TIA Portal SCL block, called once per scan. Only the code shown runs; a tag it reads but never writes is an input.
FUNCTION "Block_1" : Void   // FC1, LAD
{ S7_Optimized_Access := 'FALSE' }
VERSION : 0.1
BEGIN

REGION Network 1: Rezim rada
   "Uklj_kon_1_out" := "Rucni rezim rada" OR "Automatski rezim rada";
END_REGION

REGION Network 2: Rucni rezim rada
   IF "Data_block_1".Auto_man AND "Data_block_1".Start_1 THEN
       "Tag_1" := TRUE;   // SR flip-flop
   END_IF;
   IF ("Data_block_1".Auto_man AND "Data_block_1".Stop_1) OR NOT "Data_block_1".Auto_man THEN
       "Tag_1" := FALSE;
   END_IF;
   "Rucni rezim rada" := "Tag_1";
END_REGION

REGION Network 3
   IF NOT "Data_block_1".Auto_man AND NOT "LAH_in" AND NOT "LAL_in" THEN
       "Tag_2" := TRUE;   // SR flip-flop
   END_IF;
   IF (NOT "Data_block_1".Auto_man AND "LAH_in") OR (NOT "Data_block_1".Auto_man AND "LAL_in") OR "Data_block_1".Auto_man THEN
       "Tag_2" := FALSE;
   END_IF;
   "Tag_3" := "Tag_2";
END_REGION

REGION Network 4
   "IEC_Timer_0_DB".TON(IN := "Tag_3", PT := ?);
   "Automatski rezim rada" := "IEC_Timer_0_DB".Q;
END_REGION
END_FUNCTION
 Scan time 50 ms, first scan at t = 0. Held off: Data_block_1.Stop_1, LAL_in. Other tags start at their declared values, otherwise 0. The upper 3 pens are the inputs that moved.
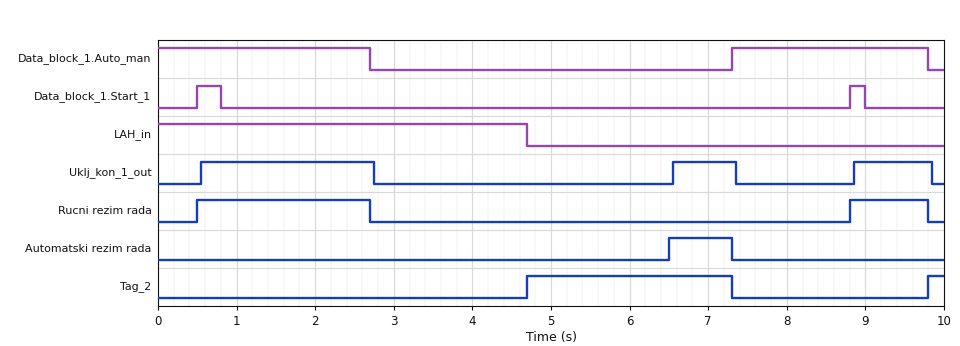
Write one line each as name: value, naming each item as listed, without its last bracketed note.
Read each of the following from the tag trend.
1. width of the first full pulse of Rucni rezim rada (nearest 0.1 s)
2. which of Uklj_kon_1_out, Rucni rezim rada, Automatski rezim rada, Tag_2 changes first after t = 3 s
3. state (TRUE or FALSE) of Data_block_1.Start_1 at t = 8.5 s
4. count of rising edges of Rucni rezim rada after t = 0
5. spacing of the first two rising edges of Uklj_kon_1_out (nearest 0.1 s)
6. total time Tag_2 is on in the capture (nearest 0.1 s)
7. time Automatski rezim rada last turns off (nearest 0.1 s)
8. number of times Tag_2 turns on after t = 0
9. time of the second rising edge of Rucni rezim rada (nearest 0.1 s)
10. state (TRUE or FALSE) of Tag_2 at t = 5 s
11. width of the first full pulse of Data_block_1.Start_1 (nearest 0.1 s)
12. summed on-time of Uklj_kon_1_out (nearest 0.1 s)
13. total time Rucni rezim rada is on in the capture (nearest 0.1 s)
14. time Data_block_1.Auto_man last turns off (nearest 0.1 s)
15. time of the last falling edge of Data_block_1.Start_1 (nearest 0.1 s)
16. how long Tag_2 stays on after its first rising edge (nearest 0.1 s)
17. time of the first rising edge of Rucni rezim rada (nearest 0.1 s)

width of the first full pulse of Rucni rezim rada: 2.2 s
which of Uklj_kon_1_out, Rucni rezim rada, Automatski rezim rada, Tag_2 changes first after t = 3 s: Tag_2
state (TRUE or FALSE) of Data_block_1.Start_1 at t = 8.5 s: FALSE
count of rising edges of Rucni rezim rada after t = 0: 2
spacing of the first two rising edges of Uklj_kon_1_out: 6.0 s
total time Tag_2 is on in the capture: 2.8 s
time Automatski rezim rada last turns off: 7.3 s
number of times Tag_2 turns on after t = 0: 2
time of the second rising edge of Rucni rezim rada: 8.8 s
state (TRUE or FALSE) of Tag_2 at t = 5 s: TRUE
width of the first full pulse of Data_block_1.Start_1: 0.3 s
summed on-time of Uklj_kon_1_out: 4.0 s
total time Rucni rezim rada is on in the capture: 3.2 s
time Data_block_1.Auto_man last turns off: 9.8 s
time of the last falling edge of Data_block_1.Start_1: 9.0 s
how long Tag_2 stays on after its first rising edge: 2.6 s
time of the first rising edge of Rucni rezim rada: 0.5 s
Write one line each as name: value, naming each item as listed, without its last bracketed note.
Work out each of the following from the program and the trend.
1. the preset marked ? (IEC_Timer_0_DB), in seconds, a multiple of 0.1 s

the preset marked ? (IEC_Timer_0_DB), in seconds, a multiple of 0.1 s: 1.8 s
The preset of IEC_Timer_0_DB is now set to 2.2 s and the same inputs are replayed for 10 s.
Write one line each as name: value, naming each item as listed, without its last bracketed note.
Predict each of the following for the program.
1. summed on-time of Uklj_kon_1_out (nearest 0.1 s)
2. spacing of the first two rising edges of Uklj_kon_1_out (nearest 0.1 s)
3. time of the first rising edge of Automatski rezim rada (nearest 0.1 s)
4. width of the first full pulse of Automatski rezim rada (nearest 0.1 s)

summed on-time of Uklj_kon_1_out: 3.6 s
spacing of the first two rising edges of Uklj_kon_1_out: 6.4 s
time of the first rising edge of Automatski rezim rada: 6.9 s
width of the first full pulse of Automatski rezim rada: 0.4 s
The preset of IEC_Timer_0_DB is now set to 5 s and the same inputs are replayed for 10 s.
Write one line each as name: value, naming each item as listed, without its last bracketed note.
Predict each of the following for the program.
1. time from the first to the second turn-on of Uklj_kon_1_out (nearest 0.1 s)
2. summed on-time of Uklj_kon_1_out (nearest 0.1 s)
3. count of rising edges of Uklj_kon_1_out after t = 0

time from the first to the second turn-on of Uklj_kon_1_out: 8.3 s
summed on-time of Uklj_kon_1_out: 3.2 s
count of rising edges of Uklj_kon_1_out after t = 0: 2
